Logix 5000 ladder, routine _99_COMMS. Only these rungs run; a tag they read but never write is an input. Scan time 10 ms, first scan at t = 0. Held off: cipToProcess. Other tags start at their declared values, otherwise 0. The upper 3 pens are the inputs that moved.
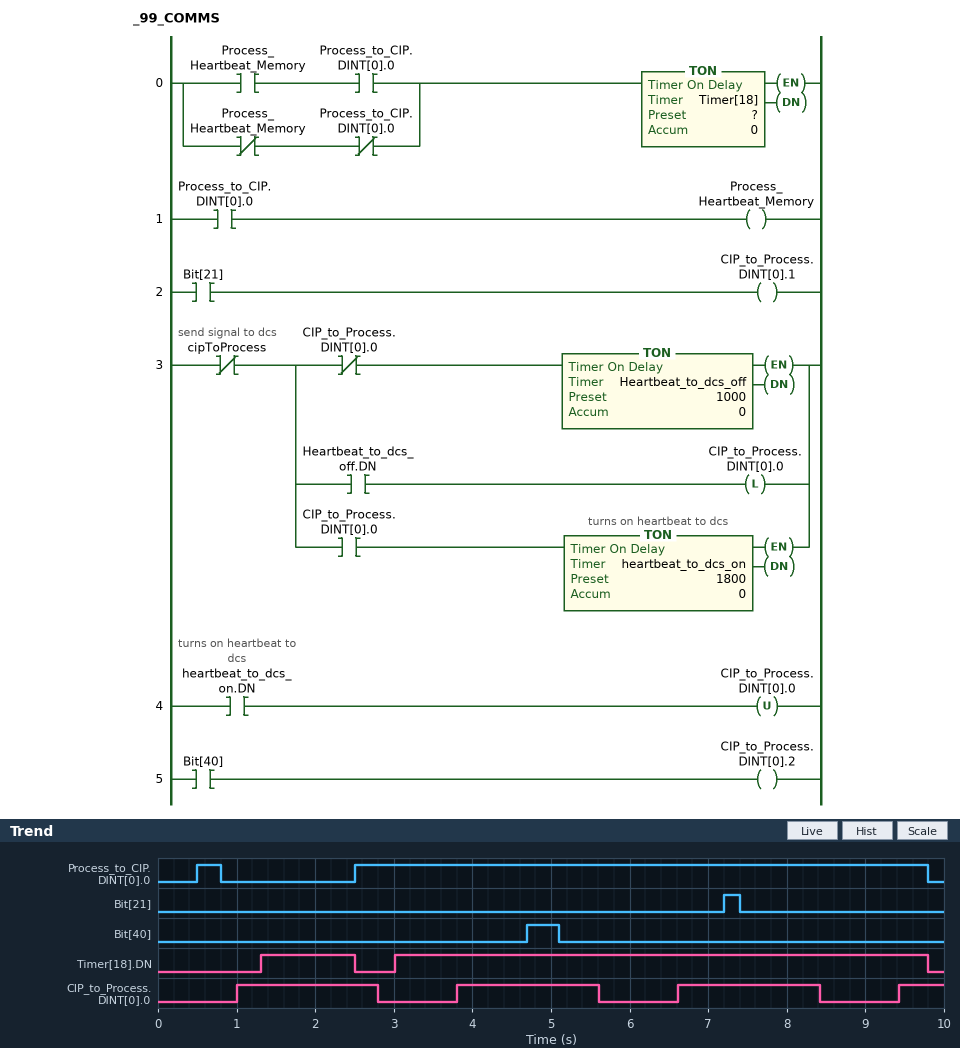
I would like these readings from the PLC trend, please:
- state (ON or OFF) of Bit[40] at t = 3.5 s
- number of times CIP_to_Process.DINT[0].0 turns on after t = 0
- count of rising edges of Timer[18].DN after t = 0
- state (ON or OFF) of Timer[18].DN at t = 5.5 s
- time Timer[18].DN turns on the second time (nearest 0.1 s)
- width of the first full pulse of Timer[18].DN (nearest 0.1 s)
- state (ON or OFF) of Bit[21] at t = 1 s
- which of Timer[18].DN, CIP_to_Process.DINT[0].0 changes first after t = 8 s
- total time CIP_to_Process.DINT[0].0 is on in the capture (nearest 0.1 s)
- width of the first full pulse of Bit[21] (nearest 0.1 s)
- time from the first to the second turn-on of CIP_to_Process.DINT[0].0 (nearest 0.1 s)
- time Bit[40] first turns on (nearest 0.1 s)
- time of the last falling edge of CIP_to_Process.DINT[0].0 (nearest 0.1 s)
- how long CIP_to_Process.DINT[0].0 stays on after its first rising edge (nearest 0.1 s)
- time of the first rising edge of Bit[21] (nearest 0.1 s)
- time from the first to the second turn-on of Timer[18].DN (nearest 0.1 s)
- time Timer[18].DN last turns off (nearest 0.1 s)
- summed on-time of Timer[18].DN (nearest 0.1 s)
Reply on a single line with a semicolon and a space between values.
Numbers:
OFF; 4; 2; ON; 3.0 s; 1.2 s; OFF; CIP_to_Process.DINT[0].0; 6.0 s; 0.2 s; 2.8 s; 4.7 s; 8.4 s; 1.8 s; 7.2 s; 1.7 s; 9.8 s; 8.0 s
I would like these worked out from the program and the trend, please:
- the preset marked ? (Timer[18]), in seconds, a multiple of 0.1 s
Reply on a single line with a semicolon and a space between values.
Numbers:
0.5 s
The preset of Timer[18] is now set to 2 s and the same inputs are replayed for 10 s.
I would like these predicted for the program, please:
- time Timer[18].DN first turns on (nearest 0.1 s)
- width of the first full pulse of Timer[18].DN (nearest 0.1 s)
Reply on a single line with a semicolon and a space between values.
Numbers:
4.5 s; 5.3 s
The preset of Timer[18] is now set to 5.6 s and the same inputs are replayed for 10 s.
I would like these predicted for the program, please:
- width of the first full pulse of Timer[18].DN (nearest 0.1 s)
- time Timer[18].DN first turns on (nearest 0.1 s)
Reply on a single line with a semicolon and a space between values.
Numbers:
1.7 s; 8.1 s
